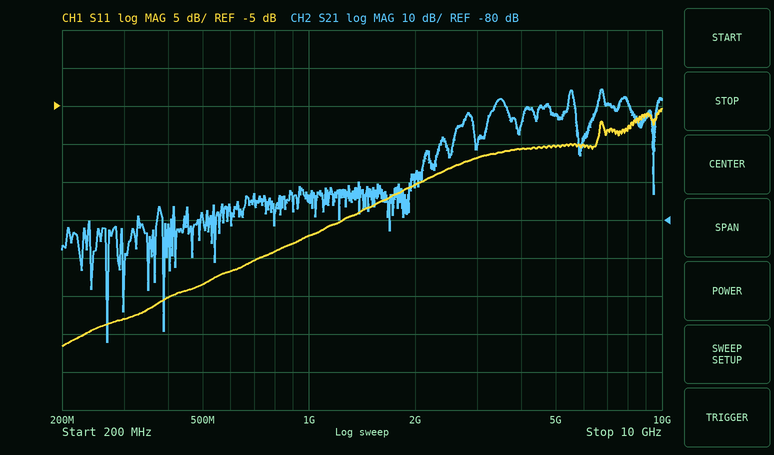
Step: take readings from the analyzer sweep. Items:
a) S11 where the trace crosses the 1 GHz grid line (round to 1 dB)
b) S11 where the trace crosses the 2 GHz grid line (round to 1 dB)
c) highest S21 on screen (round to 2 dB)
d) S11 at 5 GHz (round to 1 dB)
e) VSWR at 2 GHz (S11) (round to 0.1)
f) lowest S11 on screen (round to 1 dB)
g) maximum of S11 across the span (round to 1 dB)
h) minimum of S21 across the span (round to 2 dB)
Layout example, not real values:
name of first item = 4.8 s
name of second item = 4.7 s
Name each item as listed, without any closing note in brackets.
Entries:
S11 where the trace crosses the 1 GHz grid line = -22 dB
S11 where the trace crosses the 2 GHz grid line = -15 dB
highest S21 on screen = -46 dB
S11 at 5 GHz = -10 dB
VSWR at 2 GHz (S11) = 1.4
lowest S11 on screen = -37 dB
maximum of S11 across the span = -5 dB
minimum of S21 across the span = -112 dB
